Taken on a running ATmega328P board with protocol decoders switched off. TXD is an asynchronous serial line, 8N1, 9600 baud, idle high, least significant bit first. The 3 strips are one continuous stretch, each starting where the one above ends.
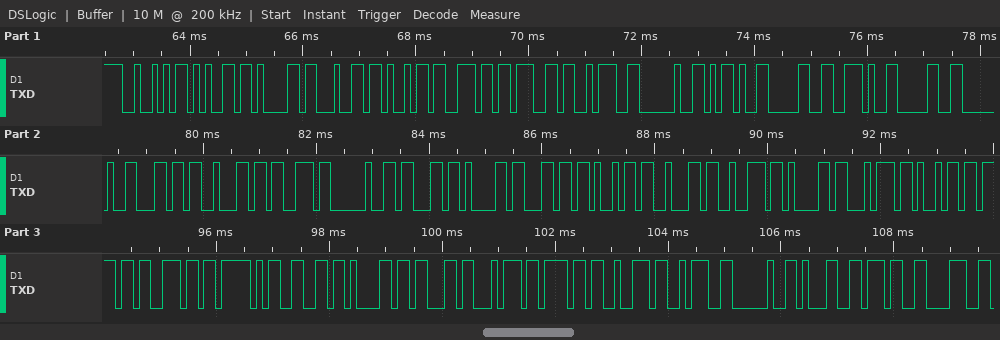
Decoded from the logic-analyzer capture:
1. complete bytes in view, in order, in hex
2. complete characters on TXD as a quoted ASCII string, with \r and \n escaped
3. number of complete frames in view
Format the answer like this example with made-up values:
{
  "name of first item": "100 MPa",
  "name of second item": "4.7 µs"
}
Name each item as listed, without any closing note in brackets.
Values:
{
  "complete bytes in view, in order, in hex": "52 65 61 64 69 6E 67 3A 20 2D 30 2E 30 20 6C 62 73 20 63 61 6C 69 62 72 61 74 69 6F 6E 5F 66 61 63 74 6F 72 3A 20 31 37 38",
  "complete characters on TXD as a quoted ASCII string, with \\r and \\n escaped": "\"Reading: -0.0 lbs calibration_factor: 178\"",
  "number of complete frames in view": "41"
}
